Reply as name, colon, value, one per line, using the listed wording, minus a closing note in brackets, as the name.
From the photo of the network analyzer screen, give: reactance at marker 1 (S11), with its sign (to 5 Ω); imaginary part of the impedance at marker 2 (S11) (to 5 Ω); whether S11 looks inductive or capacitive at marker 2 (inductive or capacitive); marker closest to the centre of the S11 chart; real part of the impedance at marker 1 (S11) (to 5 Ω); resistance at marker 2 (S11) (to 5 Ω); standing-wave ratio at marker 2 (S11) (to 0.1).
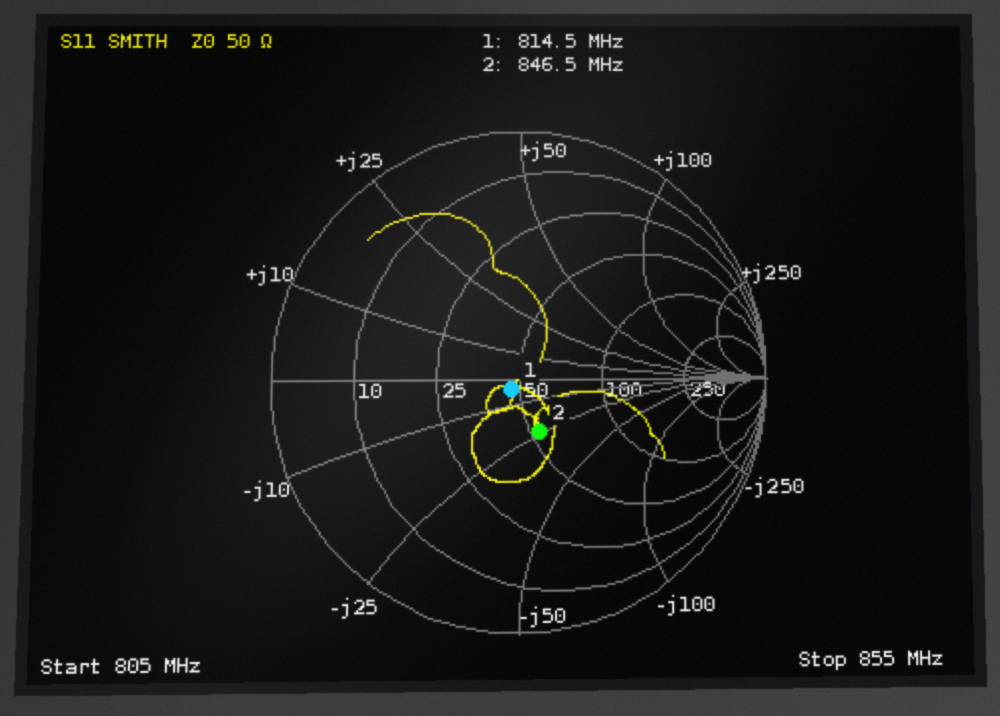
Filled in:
reactance at marker 1 (S11), with its sign: -5 Ω
imaginary part of the impedance at marker 2 (S11): -25 Ω
whether S11 looks inductive or capacitive at marker 2: capacitive
marker closest to the centre of the S11 chart: marker 1
real part of the impedance at marker 1 (S11): 45 Ω
resistance at marker 2 (S11): 55 Ω
standing-wave ratio at marker 2 (S11): 1.6
